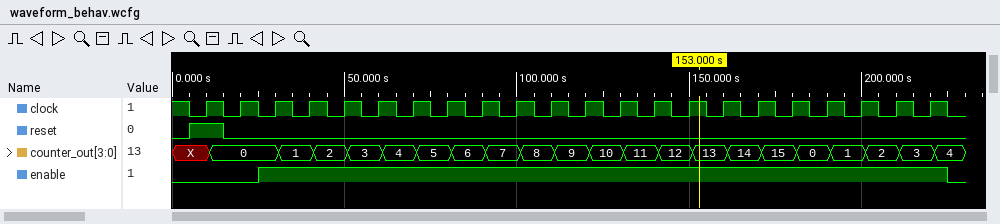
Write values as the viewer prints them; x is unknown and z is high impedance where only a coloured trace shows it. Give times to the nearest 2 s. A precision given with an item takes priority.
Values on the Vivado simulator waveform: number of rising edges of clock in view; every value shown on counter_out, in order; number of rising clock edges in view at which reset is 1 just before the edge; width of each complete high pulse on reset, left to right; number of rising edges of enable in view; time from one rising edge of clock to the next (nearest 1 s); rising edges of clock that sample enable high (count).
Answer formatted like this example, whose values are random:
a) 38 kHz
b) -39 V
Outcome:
a) 22
b) X, 0, 1, 2, 3, 4, 5, 6, 7, 8, 9, 10, 11, 12, 13, 14, 15, 0, 1, 2, 3, 4
c) 1
d) 10 s
e) 1
f) 10 s
g) 20
